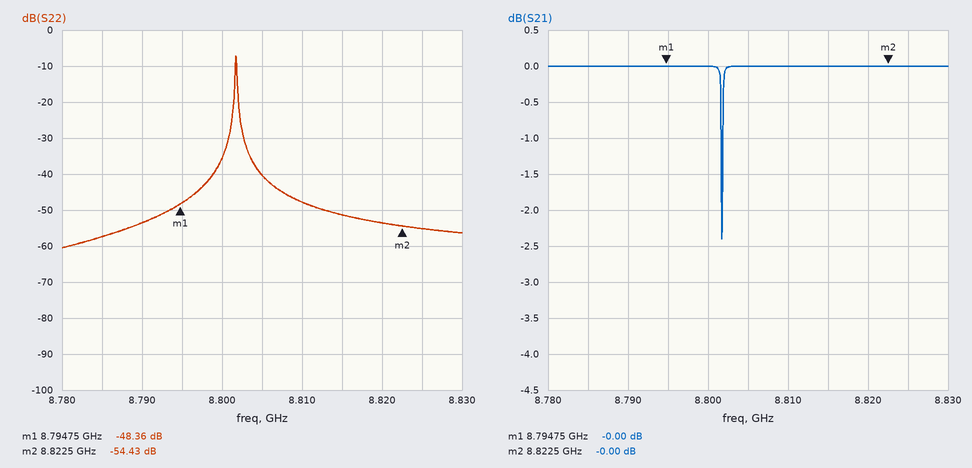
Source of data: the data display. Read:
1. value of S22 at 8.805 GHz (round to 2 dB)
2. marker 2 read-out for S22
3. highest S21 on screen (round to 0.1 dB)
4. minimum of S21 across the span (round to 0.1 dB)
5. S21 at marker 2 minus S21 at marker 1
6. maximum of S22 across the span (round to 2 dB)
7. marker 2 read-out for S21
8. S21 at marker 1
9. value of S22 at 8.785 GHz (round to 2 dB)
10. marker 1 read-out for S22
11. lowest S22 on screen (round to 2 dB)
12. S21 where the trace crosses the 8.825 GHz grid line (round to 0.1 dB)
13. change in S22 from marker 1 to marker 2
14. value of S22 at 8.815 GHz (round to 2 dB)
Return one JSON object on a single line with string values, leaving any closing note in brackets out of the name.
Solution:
{"value of S22 at 8.805 GHz": "-40 dB", "marker 2 read-out for S22": "-54.43 dB", "highest S21 on screen": "0.0 dB", "minimum of S21 across the span": "-2.4 dB", "S21 at marker 2 minus S21 at marker 1": "0.00 dB", "maximum of S22 across the span": "-8 dB", "marker 2 read-out for S21": "-0.00 dB", "S21 at marker 1": "-0.00 dB", "value of S22 at 8.785 GHz": "-58 dB", "marker 1 read-out for S22": "-48.36 dB", "lowest S22 on screen": "-60 dB", "S21 where the trace crosses the 8.825 GHz grid line": "0.0 dB", "change in S22 from marker 1 to marker 2": "-6.07 dB", "value of S22 at 8.815 GHz": "-52 dB"}
